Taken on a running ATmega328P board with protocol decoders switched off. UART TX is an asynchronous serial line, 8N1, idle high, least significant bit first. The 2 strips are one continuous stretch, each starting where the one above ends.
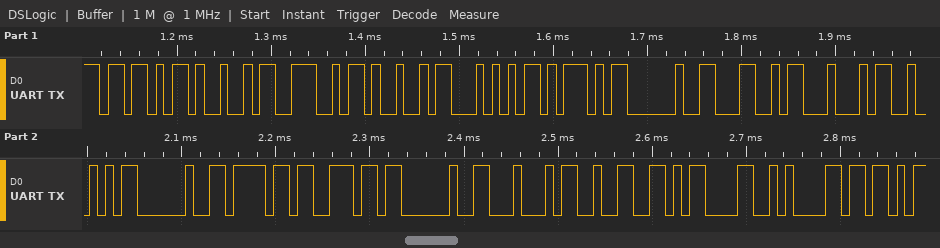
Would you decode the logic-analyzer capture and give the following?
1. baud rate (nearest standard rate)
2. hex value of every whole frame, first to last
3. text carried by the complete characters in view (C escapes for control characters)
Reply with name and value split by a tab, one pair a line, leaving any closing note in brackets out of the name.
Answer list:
baud rate	115200 baud
hex value of every whole frame, first to last	5B 49 4E 49 54 5D 20 4C 44 52 20 6F 6E 20 44 32 0D 0A 5B
text carried by the complete characters in view	"[INIT] LDR on D2\r\n["
